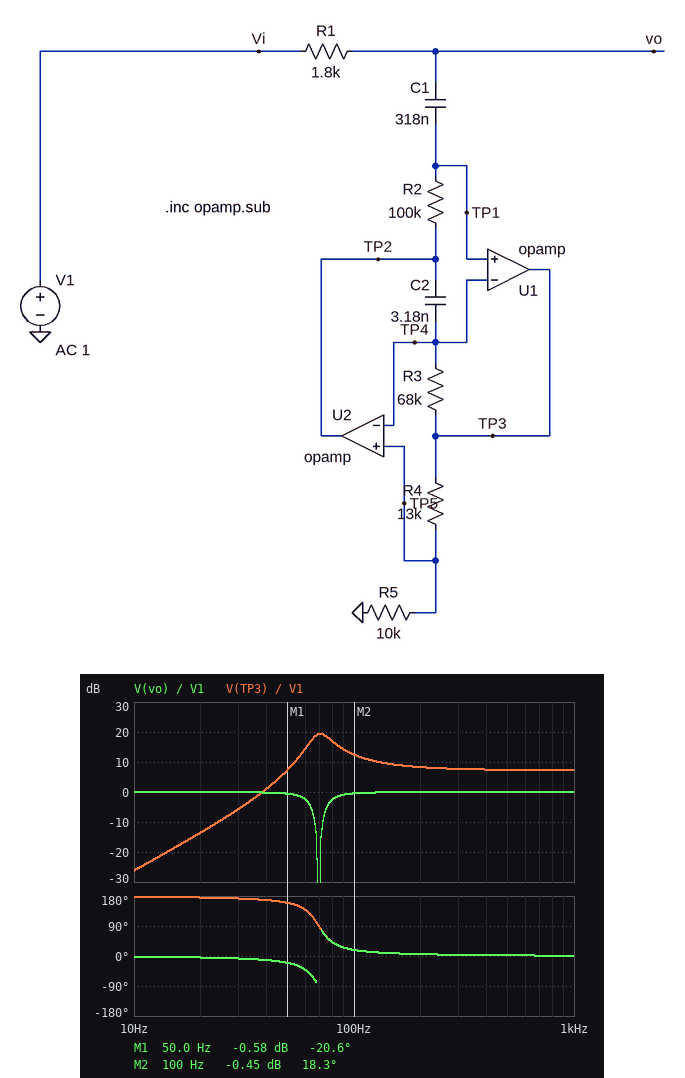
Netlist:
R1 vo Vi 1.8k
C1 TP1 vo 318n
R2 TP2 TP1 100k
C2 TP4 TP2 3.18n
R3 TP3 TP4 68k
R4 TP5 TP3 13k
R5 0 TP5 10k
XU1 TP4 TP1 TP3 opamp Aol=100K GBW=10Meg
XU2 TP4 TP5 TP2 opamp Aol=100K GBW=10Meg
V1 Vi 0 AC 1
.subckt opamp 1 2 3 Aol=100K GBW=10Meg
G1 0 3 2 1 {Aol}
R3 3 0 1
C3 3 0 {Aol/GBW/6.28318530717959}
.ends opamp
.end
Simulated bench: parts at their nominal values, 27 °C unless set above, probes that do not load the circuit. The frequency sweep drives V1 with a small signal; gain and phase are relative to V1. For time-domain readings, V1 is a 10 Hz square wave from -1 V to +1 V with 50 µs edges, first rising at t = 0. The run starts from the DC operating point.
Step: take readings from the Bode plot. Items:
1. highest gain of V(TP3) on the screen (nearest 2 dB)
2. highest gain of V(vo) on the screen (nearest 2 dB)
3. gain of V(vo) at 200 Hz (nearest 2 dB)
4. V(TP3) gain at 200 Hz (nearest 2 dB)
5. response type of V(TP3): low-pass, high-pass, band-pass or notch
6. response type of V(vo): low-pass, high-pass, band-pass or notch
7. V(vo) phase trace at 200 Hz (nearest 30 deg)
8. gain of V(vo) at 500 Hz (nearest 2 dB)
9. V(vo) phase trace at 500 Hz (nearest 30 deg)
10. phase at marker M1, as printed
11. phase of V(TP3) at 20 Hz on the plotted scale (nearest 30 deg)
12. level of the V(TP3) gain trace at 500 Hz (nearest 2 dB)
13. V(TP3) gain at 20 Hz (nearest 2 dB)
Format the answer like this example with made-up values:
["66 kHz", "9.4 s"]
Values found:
["20 dB", "0 dB", "0 dB", "8 dB", "high-pass", "notch", "0 deg", "0 dB", "0 deg", "-20.6 deg", "180 deg", "8 dB", "-14 dB"]
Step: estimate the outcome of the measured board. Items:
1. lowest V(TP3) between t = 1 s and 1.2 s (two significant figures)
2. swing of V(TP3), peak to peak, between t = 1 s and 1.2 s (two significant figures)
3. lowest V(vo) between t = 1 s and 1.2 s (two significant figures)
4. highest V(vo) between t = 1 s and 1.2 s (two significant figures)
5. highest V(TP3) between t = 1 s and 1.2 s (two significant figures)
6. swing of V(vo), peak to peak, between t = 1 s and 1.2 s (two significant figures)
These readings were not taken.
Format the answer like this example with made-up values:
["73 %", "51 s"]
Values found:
["-4.9 V", "9.8 V", "-1.3 V", "1.3 V", "4.9 V", "2.6 V"]
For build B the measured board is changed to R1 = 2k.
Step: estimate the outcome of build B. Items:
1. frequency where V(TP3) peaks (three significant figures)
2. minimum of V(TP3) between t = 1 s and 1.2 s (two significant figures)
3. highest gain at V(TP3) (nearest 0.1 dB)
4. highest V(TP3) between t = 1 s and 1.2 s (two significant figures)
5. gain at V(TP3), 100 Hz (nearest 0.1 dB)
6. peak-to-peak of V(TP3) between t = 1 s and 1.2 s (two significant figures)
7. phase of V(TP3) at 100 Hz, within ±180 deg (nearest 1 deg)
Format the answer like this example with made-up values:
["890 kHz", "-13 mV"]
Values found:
["70.6 Hz", "-4.8 V", "18.5 dB", "4.8 V", "12.3 dB", "9.6 V", "20 deg"]
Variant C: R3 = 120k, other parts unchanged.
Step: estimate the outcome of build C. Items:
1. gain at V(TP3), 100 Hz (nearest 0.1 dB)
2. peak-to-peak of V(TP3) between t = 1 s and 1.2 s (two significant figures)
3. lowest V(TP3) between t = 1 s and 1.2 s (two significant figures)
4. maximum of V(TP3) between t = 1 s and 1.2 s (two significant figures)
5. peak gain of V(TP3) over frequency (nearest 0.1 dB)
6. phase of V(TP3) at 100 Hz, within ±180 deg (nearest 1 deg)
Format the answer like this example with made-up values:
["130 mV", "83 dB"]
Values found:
["9.9 dB", "11 V", "-5.4 V", "5.4 V", "21.8 dB", "8 deg"]
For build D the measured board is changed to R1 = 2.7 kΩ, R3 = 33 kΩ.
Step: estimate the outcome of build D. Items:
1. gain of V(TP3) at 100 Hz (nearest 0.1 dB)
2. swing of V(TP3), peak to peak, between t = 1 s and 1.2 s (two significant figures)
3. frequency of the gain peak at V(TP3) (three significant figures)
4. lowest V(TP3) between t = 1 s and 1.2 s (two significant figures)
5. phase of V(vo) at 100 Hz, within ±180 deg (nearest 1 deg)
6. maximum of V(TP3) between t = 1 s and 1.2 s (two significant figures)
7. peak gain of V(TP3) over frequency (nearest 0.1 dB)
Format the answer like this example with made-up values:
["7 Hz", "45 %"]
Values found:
["12.7 dB", "9.1 V", "107 Hz", "-4.6 V", "87 deg", "4.6 V", "13.0 dB"]
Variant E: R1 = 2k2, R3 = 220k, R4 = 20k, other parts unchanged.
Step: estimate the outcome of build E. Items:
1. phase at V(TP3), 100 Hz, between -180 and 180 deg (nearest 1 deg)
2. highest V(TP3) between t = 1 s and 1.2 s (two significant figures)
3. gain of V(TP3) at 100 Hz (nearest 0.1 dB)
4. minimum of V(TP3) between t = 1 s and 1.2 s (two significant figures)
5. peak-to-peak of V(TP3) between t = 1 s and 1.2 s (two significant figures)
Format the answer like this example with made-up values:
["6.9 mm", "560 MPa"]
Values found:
["7 deg", "6.9 V", "11.7 dB", "-6.9 V", "14 V"]
